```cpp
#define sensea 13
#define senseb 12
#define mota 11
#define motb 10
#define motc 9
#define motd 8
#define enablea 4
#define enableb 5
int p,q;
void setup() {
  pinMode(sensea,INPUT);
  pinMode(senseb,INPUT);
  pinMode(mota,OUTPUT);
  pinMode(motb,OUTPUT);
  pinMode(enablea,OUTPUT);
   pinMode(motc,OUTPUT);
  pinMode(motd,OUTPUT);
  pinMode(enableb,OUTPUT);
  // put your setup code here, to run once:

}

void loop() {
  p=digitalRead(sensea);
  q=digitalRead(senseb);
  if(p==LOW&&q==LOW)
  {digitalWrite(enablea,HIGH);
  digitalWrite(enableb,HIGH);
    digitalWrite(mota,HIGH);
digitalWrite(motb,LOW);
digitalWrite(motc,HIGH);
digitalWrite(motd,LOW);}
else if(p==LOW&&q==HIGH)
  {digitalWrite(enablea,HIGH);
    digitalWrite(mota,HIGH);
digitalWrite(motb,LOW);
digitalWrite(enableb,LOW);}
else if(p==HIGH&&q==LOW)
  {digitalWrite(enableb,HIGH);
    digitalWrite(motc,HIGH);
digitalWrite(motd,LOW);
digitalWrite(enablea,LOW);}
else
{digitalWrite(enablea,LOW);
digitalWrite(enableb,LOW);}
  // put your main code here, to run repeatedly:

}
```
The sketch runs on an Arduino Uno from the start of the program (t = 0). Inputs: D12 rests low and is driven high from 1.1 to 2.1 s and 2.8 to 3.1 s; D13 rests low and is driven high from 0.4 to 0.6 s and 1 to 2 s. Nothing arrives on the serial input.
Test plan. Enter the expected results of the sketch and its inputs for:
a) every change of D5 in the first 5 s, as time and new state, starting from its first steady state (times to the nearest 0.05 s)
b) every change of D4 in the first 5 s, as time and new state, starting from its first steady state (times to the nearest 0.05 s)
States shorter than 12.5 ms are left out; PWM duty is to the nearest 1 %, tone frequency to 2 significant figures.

0 s high; 1.1 s low; 2.1 s high; 2.8 s low; 3.1 s high
0 s high; 0.4 s low; 0.6 s high; 1 s low; 2 s high
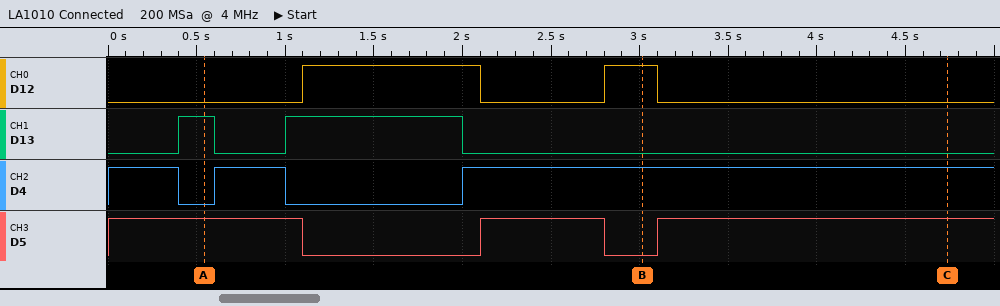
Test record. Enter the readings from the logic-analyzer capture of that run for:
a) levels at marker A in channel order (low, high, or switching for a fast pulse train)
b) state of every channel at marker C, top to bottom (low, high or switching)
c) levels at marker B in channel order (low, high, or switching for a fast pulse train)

D12 low, D13 high, D4 low, D5 high
D12 low, D13 low, D4 high, D5 high
D12 high, D13 low, D4 high, D5 low
